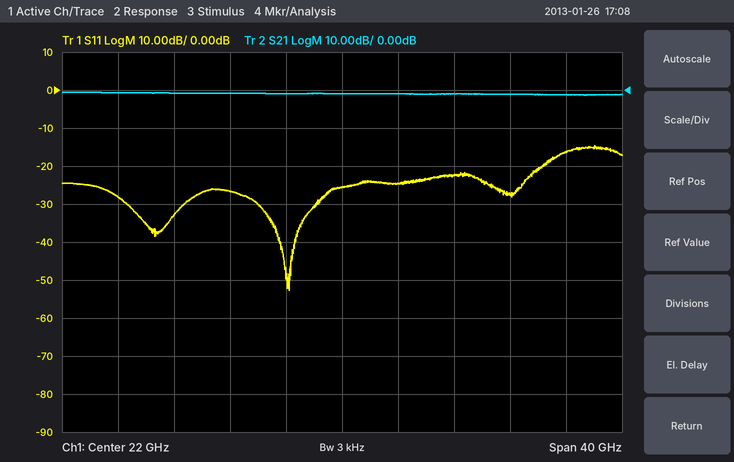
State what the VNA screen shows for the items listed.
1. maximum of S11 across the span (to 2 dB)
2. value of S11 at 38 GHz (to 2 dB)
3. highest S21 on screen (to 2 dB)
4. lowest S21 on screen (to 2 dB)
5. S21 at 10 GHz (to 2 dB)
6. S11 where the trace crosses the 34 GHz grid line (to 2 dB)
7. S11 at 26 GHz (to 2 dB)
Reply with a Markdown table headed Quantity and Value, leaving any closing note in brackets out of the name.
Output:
| Quantity | Value |
|---|---|
| maximum of S11 across the span | -14 dB |
| value of S11 at 38 GHz | -16 dB |
| highest S21 on screen | 0 dB |
| lowest S21 on screen | -2 dB |
| S21 at 10 GHz | 0 dB |
| S11 where the trace crosses the 34 GHz grid line | -28 dB |
| S11 at 26 GHz | -24 dB |
